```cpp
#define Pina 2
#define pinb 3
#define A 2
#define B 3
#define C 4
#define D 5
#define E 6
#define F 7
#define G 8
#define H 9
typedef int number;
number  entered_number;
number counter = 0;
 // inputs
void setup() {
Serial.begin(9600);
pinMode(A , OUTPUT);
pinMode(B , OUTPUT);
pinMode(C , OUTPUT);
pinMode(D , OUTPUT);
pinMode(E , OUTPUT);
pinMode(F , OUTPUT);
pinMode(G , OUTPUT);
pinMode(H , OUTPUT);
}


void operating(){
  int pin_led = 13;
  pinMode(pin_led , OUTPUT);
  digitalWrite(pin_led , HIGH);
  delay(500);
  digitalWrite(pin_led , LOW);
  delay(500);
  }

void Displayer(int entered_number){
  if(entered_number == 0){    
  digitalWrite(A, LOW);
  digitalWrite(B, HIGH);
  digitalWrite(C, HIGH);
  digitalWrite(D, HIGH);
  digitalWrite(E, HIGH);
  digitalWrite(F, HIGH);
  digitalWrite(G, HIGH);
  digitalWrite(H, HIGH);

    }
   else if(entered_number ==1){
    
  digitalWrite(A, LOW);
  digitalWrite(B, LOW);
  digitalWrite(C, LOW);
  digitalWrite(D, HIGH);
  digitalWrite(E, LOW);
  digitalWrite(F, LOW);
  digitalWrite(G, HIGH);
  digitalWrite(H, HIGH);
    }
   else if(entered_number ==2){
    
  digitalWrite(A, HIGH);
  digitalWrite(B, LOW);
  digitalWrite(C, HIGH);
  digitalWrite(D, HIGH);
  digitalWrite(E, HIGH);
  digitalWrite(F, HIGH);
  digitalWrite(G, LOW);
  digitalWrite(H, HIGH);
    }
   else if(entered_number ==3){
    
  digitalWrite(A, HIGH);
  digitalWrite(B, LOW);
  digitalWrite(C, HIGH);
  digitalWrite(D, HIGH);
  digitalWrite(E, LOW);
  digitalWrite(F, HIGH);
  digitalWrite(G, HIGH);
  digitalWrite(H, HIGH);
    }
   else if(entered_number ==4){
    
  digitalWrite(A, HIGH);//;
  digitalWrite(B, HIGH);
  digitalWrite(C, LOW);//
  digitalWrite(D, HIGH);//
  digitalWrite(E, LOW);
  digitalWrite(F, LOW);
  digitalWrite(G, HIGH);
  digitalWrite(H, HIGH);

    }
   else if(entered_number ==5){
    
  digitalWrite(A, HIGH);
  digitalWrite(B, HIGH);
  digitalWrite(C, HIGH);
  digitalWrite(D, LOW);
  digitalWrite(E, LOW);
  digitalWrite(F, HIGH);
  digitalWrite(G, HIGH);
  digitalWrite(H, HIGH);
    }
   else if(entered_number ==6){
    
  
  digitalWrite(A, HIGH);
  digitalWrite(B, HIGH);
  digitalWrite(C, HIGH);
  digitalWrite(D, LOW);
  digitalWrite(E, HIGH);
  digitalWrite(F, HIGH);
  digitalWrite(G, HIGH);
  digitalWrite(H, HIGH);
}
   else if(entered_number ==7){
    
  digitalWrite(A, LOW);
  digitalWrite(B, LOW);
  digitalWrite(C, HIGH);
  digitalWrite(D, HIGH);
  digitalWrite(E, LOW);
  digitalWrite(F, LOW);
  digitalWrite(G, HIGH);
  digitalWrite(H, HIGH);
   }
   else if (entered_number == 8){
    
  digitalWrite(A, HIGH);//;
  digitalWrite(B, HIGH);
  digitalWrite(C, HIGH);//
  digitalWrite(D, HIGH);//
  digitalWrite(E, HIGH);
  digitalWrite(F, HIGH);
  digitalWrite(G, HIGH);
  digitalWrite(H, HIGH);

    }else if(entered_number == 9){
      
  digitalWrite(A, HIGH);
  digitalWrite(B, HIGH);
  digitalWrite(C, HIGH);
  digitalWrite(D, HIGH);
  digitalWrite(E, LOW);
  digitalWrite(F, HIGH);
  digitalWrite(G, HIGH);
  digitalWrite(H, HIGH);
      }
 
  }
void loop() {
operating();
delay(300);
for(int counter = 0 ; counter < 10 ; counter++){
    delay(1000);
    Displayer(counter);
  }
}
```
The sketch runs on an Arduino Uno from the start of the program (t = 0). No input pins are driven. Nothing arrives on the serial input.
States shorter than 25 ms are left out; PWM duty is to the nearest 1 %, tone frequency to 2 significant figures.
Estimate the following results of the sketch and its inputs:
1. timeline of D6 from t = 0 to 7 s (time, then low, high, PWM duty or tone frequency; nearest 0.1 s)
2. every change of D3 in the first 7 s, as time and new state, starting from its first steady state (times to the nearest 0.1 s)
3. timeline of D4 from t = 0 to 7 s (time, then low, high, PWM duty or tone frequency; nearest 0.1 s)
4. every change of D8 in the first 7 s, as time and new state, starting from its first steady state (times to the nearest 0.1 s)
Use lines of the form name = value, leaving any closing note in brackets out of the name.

timeline of D6 from t = 0 to 7 s = 0 s low; 2.3 s high; 3.3 s low; 4.3 s high; 5.3 s low
every change of D3 in the first 7 s, as time and new state, starting from its first steady state = 0 s low; 2.3 s high; 3.3 s low; 6.3 s high
timeline of D4 from t = 0 to 7 s = 0 s low; 2.3 s high; 3.3 s low; 4.3 s high; 6.3 s low
every change of D8 in the first 7 s, as time and new state, starting from its first steady state = 0 s low; 2.3 s high; 4.3 s low; 5.3 s high
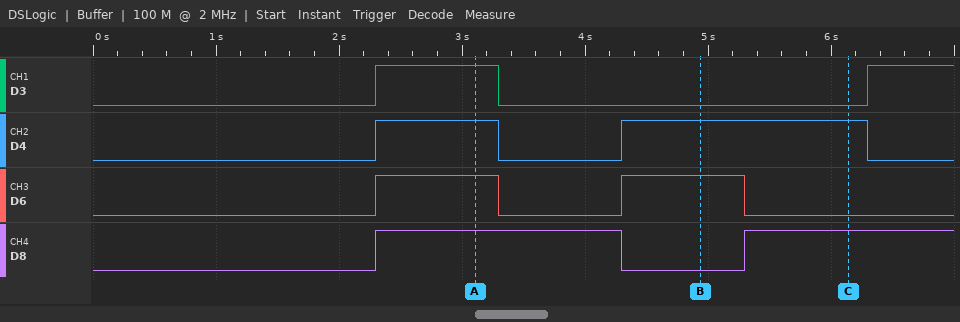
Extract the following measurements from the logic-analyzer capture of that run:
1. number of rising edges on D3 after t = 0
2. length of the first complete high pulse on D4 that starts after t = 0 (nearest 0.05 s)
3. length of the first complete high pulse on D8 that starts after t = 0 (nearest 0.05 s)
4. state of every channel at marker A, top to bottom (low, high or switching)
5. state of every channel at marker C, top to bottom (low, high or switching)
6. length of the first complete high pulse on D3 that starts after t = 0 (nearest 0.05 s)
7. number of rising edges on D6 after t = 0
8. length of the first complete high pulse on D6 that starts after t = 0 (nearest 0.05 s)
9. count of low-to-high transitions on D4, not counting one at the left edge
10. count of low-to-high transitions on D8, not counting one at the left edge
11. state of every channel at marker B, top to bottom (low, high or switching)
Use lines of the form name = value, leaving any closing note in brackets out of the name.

number of rising edges on D3 after t = 0 = 2
length of the first complete high pulse on D4 that starts after t = 0 = 1.00 s
length of the first complete high pulse on D8 that starts after t = 0 = 2.00 s
state of every channel at marker A, top to bottom = D3 high, D4 high, D6 high, D8 high
state of every channel at marker C, top to bottom = D3 low, D4 high, D6 low, D8 high
length of the first complete high pulse on D3 that starts after t = 0 = 1.00 s
number of rising edges on D6 after t = 0 = 2
length of the first complete high pulse on D6 that starts after t = 0 = 1.00 s
count of low-to-high transitions on D4, not counting one at the left edge = 2
count of low-to-high transitions on D8, not counting one at the left edge = 2
state of every channel at marker B, top to bottom = D3 low, D4 high, D6 high, D8 low
